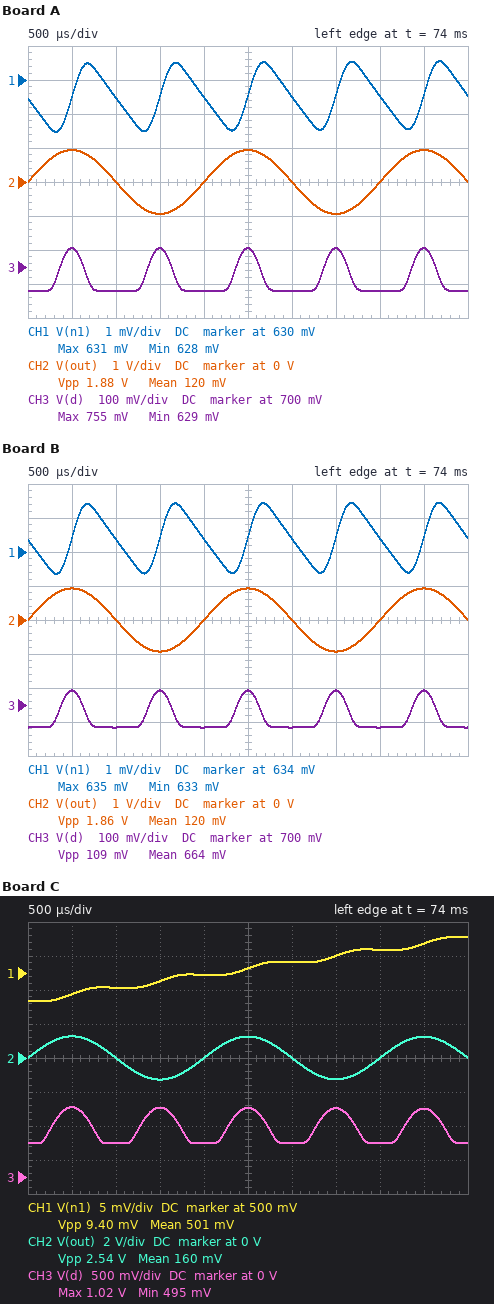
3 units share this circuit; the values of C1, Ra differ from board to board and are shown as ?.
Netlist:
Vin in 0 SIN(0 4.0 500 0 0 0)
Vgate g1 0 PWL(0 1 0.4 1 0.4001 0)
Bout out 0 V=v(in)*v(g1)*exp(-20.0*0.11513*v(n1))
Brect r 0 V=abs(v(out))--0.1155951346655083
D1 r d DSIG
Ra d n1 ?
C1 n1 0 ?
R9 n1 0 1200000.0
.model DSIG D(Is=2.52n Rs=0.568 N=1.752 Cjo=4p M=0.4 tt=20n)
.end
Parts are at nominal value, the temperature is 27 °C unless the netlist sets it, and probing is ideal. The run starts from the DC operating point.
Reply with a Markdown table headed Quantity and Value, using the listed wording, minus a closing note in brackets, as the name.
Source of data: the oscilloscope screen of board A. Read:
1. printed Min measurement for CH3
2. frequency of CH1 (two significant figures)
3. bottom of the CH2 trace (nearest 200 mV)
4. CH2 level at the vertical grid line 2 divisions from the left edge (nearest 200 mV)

| Quantity | Value |
|---|---|
| printed Min measurement for CH3 | 629 mV |
| frequency of CH1 | 1.0 kHz |
| bottom of the CH2 trace | -1.0 V |
| CH2 level at the vertical grid line 2 divisions from the left edge | 0 V |
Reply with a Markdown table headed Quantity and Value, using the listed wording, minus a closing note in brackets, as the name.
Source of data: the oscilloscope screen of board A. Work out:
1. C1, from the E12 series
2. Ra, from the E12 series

| Quantity | Value |
|---|---|
| C1, from the E12 series | 150 nF |
| Ra, from the E12 series | 68 kΩ |
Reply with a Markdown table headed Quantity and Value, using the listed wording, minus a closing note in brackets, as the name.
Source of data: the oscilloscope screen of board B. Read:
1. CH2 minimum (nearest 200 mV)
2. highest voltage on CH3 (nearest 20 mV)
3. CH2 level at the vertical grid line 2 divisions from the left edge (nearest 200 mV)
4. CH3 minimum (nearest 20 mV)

| Quantity | Value |
|---|---|
| CH2 minimum | -1.0 V |
| highest voltage on CH3 | 740 mV |
| CH2 level at the vertical grid line 2 divisions from the left edge | 0 V |
| CH3 minimum | 640 mV |
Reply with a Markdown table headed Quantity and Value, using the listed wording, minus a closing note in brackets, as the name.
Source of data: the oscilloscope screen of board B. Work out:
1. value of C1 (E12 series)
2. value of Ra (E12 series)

| Quantity | Value |
|---|---|
| value of C1 | 150 nF |
| value of Ra | 56 kΩ |
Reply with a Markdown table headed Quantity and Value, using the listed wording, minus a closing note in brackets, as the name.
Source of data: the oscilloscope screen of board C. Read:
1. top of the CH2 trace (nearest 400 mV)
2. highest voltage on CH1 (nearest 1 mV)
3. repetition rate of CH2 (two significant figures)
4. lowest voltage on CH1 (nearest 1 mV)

| Quantity | Value |
|---|---|
| top of the CH2 trace | 1.2 V |
| highest voltage on CH1 | 505 mV |
| repetition rate of CH2 | 500 Hz |
| lowest voltage on CH1 | 496 mV |
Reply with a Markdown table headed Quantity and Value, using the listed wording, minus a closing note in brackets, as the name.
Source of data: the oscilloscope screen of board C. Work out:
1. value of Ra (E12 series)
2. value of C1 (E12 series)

| Quantity | Value |
|---|---|
| value of Ra | 68 kΩ |
| value of C1 | 1.5 µF |
